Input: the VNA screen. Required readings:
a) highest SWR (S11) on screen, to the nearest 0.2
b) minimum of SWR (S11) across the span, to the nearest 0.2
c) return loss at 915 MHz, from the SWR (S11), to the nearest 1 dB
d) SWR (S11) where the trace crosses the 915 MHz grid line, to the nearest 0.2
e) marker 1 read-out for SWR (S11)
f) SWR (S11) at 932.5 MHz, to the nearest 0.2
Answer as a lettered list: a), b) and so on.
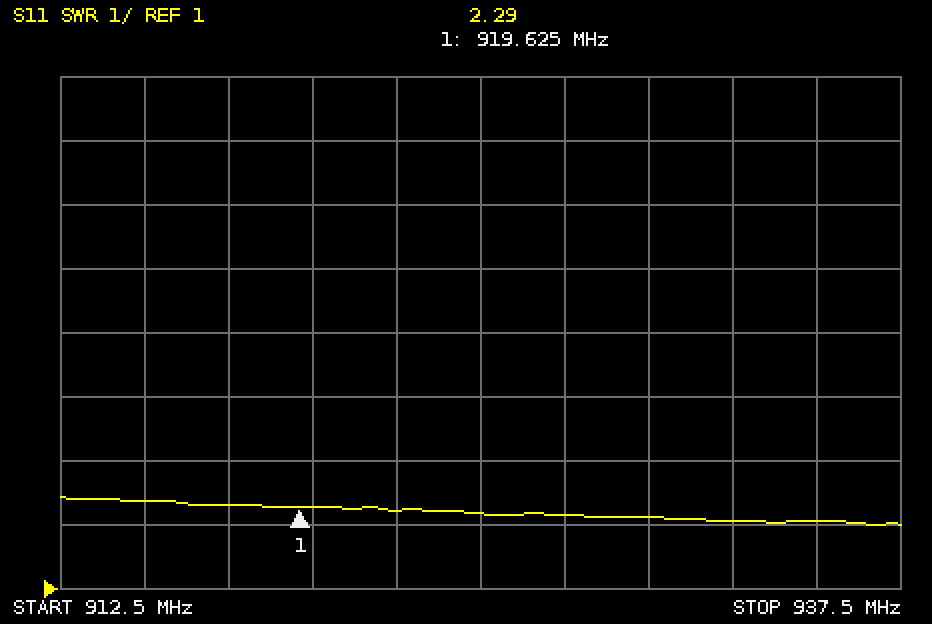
a) 2.4
b) 2.0
c) 8 dB
d) 2.4
e) 2.29
f) 2.0
